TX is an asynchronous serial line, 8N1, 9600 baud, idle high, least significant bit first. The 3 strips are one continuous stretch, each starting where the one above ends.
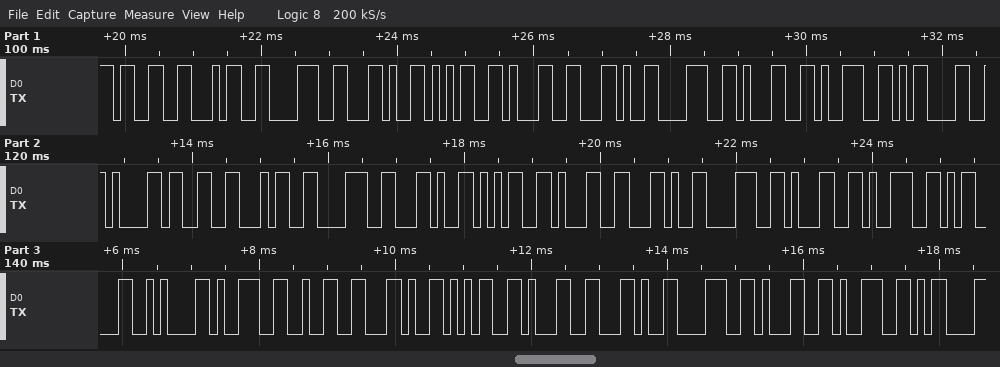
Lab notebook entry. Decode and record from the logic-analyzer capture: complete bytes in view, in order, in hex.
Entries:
33 34 38 2C 35 31 2C 38 31 39 0D 0A 33 34 38 2C 35 31 2C 38 31 39 0D 0A 39 32 2C 35 31 2C 38 31 39 0D
